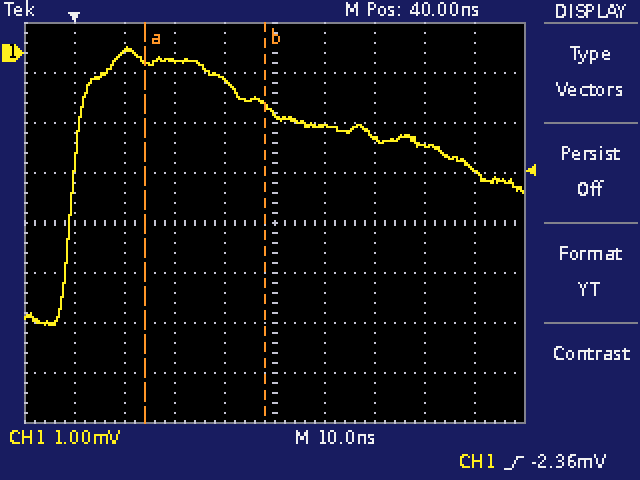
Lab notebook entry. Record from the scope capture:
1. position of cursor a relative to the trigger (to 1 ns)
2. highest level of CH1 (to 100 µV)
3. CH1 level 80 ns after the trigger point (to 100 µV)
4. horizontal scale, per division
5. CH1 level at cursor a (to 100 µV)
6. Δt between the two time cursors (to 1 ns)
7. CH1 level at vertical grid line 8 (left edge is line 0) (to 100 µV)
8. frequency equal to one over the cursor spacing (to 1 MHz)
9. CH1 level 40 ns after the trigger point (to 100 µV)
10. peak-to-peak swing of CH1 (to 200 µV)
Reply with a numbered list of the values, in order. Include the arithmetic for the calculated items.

1. +14 ns
2. 100 µV
3. -2.3 mV
4. 10 ns
5. -200 µV
6. 24 ns
7. -1.9 mV
8. 1 / 24 ns ≈ 42 MHz
9. -1.2 mV
10. 5.6 mV
